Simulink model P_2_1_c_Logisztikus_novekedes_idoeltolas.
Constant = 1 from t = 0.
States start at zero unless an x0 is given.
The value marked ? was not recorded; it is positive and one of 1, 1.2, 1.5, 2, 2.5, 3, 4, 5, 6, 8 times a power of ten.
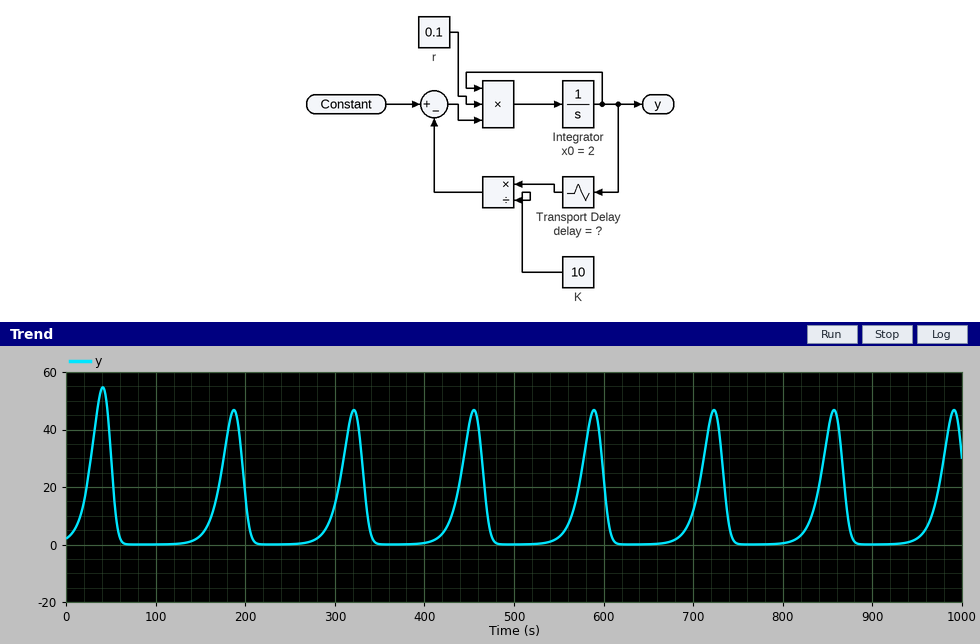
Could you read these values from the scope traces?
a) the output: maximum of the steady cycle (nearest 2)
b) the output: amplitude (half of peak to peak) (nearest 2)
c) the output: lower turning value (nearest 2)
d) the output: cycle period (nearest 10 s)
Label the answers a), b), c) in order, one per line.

a) 46
b) 24
c) 0
d) 130 s
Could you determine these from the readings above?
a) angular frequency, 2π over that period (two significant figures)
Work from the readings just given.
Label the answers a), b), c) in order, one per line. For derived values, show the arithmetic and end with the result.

a) 2π / 130 = 0.048 rad/s
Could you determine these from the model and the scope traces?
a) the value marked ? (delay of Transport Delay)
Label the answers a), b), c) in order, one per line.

a) 25
